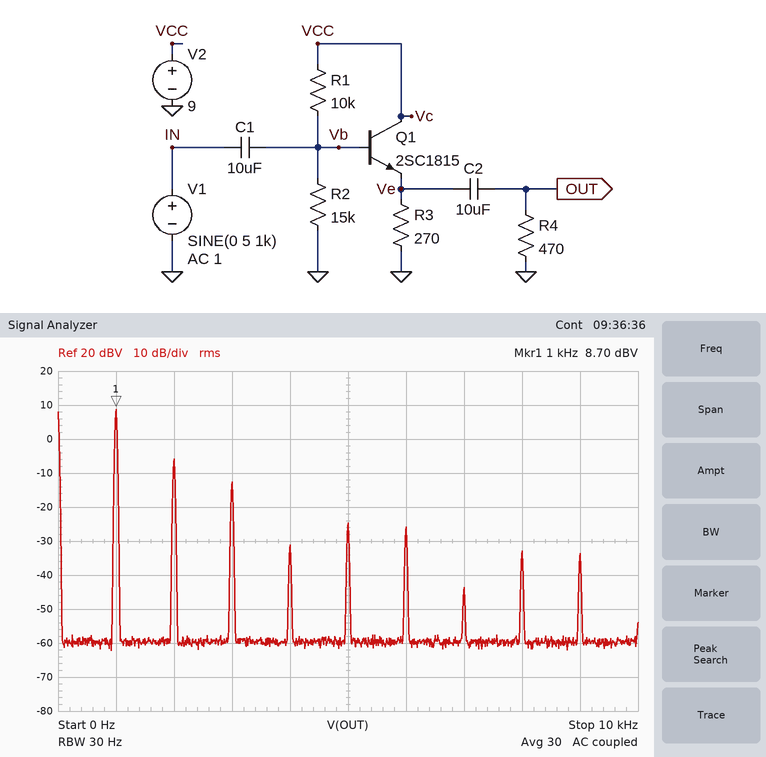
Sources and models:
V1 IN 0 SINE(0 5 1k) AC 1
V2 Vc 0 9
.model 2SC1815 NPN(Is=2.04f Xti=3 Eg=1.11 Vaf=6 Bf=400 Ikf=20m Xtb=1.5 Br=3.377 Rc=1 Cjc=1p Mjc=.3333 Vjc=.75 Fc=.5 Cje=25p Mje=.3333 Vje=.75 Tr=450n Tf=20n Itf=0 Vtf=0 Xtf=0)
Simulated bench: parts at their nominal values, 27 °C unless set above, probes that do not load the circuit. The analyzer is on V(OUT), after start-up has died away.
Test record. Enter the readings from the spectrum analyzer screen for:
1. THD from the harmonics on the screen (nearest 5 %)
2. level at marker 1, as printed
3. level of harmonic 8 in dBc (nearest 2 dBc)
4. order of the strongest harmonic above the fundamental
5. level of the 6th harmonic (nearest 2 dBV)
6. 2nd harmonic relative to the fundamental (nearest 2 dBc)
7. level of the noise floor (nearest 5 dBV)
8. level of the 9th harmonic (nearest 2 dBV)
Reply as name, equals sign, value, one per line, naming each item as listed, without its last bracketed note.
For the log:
THD from the harmonics on the screen = 20 %
level at marker 1, as printed = 8.70 dBV
level of harmonic 8 in dBc = -42 dBc
order of the strongest harmonic above the fundamental = 2
level of the 6th harmonic = -26 dBV
2nd harmonic relative to the fundamental = -14 dBc
level of the noise floor = -60 dBV
level of the 9th harmonic = -34 dBV
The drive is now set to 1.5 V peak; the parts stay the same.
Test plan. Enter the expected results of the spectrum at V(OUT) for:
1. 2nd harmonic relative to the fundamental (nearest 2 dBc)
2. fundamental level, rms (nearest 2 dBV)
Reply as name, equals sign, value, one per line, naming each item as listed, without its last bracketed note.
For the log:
2nd harmonic relative to the fundamental = -58 dBc
fundamental level, rms = 0 dBV
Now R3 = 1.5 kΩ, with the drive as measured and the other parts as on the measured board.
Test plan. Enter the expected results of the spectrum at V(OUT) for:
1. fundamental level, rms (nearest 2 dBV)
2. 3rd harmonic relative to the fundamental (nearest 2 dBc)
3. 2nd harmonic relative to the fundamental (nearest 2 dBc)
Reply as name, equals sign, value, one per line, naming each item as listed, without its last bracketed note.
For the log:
fundamental level, rms = 4 dBV
3rd harmonic relative to the fundamental = -30 dBc
2nd harmonic relative to the fundamental = -6 dBc
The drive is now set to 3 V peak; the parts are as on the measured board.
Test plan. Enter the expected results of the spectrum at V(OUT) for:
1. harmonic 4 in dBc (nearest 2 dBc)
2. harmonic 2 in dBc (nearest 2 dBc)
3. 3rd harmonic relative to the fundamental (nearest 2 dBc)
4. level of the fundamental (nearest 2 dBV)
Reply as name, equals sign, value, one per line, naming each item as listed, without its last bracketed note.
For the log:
harmonic 4 in dBc = -42 dBc
harmonic 2 in dBc = -38 dBc
3rd harmonic relative to the fundamental = -40 dBc
level of the fundamental = 6 dBV
